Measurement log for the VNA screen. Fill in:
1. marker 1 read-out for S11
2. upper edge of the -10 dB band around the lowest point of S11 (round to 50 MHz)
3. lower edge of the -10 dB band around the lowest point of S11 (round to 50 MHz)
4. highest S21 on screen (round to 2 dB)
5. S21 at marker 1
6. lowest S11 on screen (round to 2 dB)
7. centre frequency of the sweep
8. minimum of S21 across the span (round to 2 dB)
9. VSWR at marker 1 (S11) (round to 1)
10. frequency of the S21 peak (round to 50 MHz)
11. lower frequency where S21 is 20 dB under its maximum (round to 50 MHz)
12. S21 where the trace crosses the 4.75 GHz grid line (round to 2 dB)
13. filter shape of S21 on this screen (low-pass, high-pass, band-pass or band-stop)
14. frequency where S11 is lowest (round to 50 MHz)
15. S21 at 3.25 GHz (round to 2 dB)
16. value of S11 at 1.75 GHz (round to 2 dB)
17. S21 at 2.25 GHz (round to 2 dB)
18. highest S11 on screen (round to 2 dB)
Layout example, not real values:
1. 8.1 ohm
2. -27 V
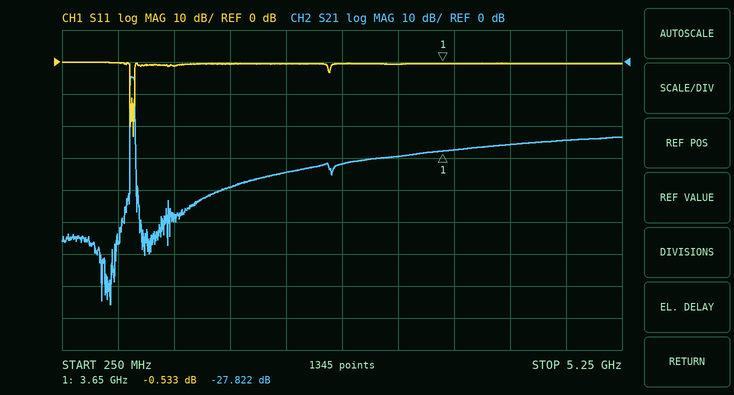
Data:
1. -0.533 dB
2. 900 MHz
3. 850 MHz
4. -4 dB
5. -27.822 dB
6. -24 dB
7. 2.75 GHz
8. -76 dB
9. 33
10. 850 MHz
11. 850 MHz
12. -24 dB
13. band-pass
14. 900 MHz
15. -30 dB
16. 0 dB
17. -34 dB
18. 0 dB
